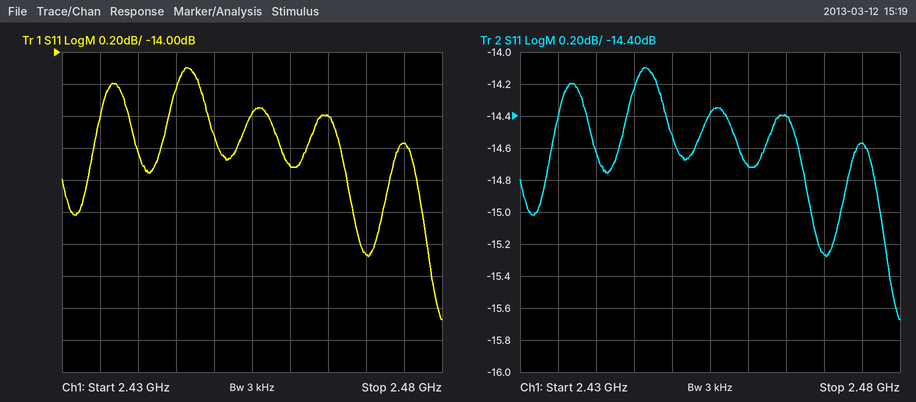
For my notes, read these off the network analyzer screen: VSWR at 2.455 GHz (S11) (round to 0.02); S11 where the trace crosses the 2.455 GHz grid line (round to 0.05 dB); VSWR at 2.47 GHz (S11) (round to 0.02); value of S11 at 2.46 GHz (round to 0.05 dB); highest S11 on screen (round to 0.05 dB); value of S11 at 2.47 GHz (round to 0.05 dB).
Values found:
1.48
-14.40 dB
1.42
-14.70 dB
-14.10 dB
-15.25 dB
